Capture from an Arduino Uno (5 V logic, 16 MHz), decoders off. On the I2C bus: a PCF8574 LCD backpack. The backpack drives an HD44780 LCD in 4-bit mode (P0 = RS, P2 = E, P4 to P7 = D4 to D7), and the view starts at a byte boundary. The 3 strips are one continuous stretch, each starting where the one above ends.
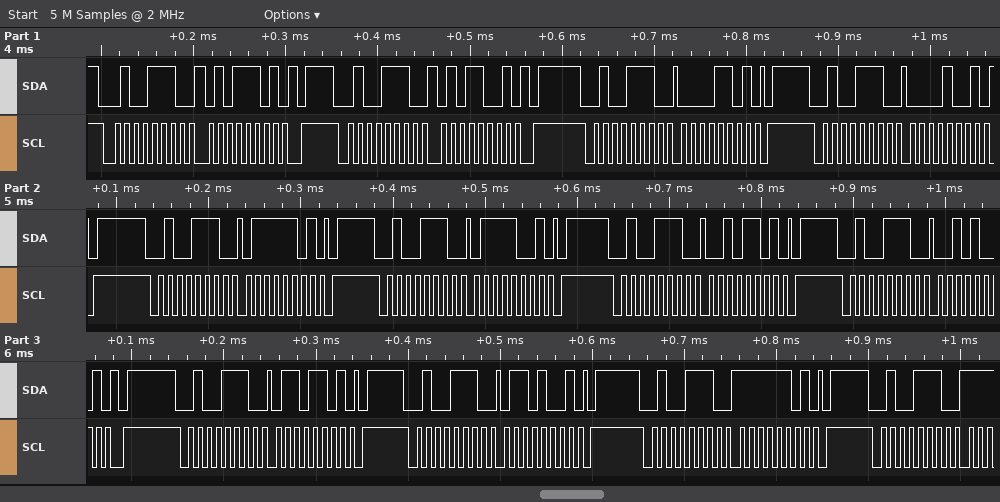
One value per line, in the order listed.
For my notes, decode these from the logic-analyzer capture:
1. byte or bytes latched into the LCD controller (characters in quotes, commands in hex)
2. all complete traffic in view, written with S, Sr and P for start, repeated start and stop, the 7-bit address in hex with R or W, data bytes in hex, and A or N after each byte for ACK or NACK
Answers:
'P' 'r'
S 27W A 5D A P S 27W A 59 A P S 27W A 0D A P S 27W A 09 A P S 27W A 7D A P S 27W A 79 A P S 27W A 2D A P S 27W A 29 A P S 27W A 6D A P S 27W A 69 A P S 27W A FD A P S 27W A
